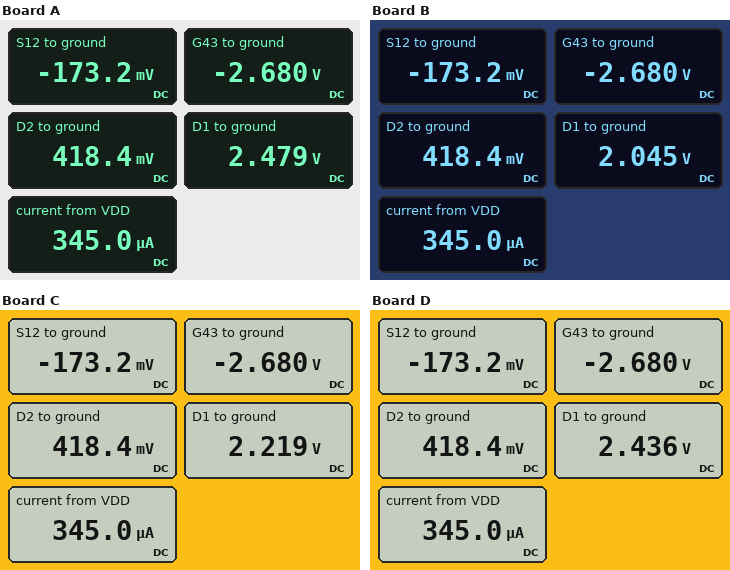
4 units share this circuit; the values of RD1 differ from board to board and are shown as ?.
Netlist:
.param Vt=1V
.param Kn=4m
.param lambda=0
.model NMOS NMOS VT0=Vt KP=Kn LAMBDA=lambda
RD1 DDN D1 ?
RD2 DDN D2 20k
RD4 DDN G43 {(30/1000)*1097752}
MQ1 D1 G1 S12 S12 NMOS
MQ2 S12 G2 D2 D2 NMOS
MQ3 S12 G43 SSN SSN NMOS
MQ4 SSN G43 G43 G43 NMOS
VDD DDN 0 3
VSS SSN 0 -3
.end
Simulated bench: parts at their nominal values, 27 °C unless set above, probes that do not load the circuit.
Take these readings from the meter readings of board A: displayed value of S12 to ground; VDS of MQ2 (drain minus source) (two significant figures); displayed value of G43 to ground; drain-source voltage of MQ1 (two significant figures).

-173.2 mV
-590 mV
-2.680 V
2.7 V
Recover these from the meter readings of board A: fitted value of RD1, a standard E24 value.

12 kΩ
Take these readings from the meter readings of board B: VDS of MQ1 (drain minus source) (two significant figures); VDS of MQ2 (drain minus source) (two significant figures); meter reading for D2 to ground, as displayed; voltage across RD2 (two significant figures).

2.2 V
-590 mV
418.4 mV
2.6 V
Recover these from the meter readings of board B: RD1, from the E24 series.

22 kΩ
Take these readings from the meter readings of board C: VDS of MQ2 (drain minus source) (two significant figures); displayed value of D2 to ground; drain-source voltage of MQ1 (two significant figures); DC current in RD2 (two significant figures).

-590 mV
418.4 mV
2.4 V
130 µA
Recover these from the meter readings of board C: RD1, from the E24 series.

18 kΩ
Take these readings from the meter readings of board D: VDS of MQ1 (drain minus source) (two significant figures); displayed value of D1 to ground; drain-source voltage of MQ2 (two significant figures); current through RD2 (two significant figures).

2.6 V
2.436 V
-590 mV
130 µA
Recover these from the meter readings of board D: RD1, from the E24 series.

13 kΩ
